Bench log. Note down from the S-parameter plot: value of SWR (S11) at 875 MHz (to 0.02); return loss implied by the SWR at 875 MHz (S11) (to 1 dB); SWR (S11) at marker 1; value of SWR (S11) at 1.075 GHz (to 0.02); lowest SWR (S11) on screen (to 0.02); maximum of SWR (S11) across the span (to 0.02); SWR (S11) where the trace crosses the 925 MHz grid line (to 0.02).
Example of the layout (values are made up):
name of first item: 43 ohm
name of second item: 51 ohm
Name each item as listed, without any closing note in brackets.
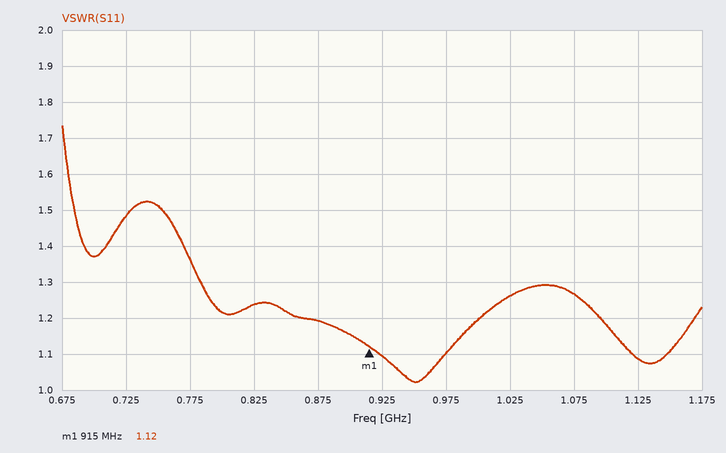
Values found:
value of SWR (S11) at 875 MHz: 1.20
return loss implied by the SWR at 875 MHz (S11): 21 dB
SWR (S11) at marker 1: 1.12
value of SWR (S11) at 1.075 GHz: 1.26
lowest SWR (S11) on screen: 1.02
maximum of SWR (S11) across the span: 1.74
SWR (S11) where the trace crosses the 925 MHz grid line: 1.10
